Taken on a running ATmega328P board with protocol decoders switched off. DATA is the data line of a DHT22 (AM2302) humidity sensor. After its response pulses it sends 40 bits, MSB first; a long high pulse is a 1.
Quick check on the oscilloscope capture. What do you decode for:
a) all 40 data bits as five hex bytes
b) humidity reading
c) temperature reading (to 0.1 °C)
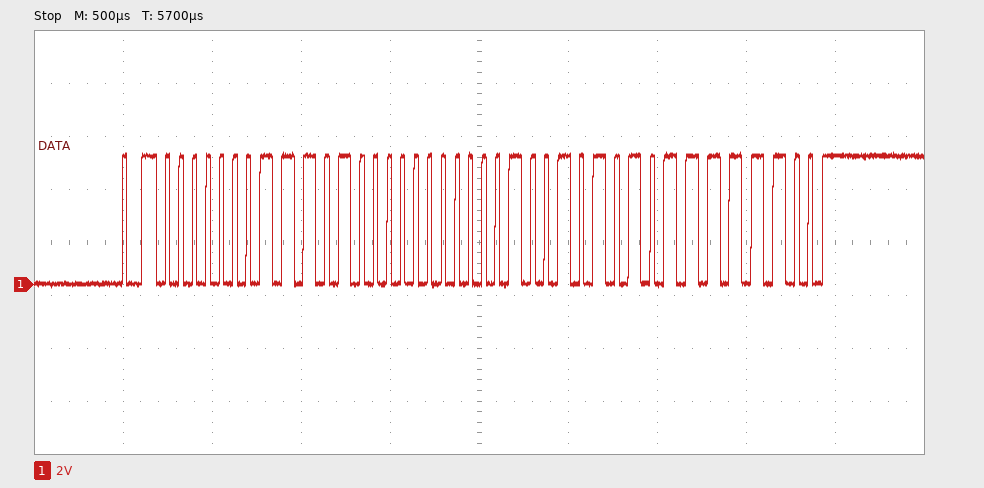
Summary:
01 D0 01 2A FC
46.4 %
29.8 °C
